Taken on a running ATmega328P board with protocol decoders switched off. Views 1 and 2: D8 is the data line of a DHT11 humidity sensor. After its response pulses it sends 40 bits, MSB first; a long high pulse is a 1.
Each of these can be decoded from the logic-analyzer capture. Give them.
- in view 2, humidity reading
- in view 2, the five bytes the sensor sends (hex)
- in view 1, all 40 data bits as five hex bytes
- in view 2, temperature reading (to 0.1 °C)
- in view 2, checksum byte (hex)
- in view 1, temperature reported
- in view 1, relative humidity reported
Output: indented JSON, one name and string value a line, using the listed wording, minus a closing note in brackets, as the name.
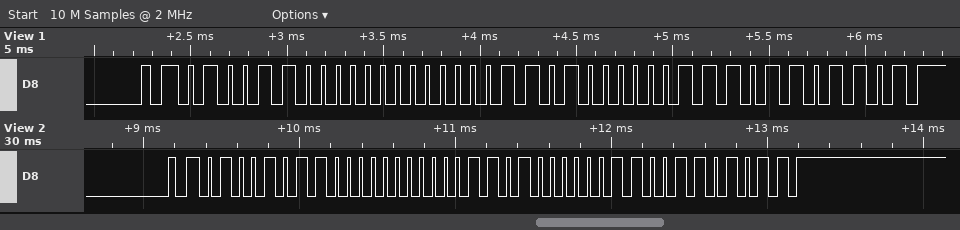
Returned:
{
  "in view 2, humidity reading": "75 %",
  "in view 2, the five bytes the sensor sends": "4B 00 1A 06 6B",
  "in view 1, all 40 data bits as five hex bytes": "4C 00 1A 07 6D",
  "in view 2, temperature reading": "26.6 °C",
  "in view 2, checksum byte": "0x6B",
  "in view 1, temperature reported": "26.7 °C",
  "in view 1, relative humidity reported": "76 %"
}
